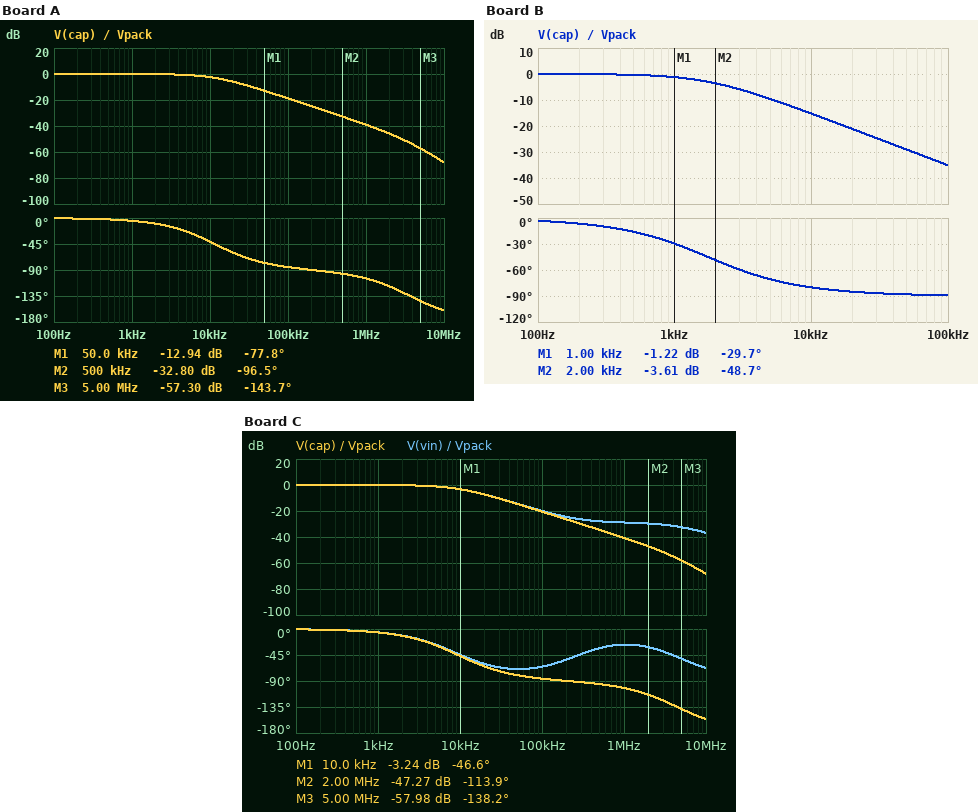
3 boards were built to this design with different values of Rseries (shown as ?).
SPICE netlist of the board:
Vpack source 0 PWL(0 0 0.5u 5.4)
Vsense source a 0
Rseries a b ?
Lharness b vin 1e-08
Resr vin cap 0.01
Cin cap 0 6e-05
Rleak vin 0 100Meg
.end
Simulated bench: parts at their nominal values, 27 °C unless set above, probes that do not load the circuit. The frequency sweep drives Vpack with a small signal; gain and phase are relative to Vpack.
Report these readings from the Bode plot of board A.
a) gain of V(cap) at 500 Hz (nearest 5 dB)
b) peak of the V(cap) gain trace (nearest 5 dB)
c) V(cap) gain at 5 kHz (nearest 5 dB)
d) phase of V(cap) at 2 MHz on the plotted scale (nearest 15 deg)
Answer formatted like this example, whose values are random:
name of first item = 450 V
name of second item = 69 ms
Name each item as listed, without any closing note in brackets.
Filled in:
gain of V(cap) at 500 Hz = 0 dB
peak of the V(cap) gain trace = 0 dB
V(cap) gain at 5 kHz = 0 dB
phase of V(cap) at 2 MHz on the plotted scale = -120 deg
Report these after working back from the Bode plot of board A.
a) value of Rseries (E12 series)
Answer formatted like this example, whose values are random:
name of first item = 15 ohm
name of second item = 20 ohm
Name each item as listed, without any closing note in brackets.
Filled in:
value of Rseries = 0.22 Ω
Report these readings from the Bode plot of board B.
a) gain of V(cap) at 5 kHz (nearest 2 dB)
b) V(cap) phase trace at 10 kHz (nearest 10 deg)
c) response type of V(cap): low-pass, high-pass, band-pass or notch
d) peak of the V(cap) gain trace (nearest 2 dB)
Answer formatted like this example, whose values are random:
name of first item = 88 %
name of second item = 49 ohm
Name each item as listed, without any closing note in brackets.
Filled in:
gain of V(cap) at 5 kHz = -10 dB
V(cap) phase trace at 10 kHz = -80 deg
response type of V(cap): low-pass, high-pass, band-pass or notch = low-pass
peak of the V(cap) gain trace = 0 dB
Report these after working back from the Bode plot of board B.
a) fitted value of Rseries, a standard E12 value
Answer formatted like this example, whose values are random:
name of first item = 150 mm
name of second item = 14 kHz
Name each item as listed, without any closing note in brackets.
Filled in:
fitted value of Rseries, a standard E12 value = 1.5 Ω
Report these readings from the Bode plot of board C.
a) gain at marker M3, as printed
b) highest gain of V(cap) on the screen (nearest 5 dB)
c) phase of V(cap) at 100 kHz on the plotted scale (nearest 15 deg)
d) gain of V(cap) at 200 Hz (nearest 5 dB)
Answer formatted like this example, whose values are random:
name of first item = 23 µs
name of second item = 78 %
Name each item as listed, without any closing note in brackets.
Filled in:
gain at marker M3, as printed = -57.98 dB
highest gain of V(cap) on the screen = 0 dB
phase of V(cap) at 100 kHz on the plotted scale = -90 deg
gain of V(cap) at 200 Hz = 0 dB
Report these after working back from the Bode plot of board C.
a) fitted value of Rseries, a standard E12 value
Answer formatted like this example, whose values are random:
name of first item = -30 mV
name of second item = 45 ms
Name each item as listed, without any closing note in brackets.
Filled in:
fitted value of Rseries, a standard E12 value = 0.27 Ω
